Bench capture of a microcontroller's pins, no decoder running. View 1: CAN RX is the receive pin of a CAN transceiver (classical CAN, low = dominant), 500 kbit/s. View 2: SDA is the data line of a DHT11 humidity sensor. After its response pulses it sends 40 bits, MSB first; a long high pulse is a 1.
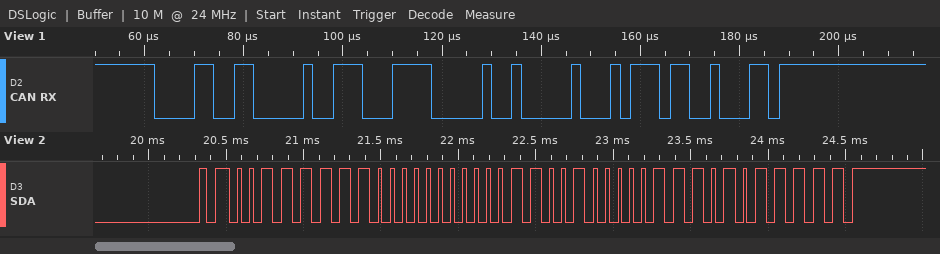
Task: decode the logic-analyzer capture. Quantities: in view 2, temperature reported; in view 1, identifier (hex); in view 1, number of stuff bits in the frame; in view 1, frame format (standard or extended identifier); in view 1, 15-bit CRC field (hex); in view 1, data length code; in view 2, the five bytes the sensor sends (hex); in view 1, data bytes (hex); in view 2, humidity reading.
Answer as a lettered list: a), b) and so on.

a) 25.7 °C
b) 0x0CC
c) 3
d) standard
e) 0x5D91
f) 3
g) 3F 00 19 07 5F
h) 8F 01 00
i) 63 %
